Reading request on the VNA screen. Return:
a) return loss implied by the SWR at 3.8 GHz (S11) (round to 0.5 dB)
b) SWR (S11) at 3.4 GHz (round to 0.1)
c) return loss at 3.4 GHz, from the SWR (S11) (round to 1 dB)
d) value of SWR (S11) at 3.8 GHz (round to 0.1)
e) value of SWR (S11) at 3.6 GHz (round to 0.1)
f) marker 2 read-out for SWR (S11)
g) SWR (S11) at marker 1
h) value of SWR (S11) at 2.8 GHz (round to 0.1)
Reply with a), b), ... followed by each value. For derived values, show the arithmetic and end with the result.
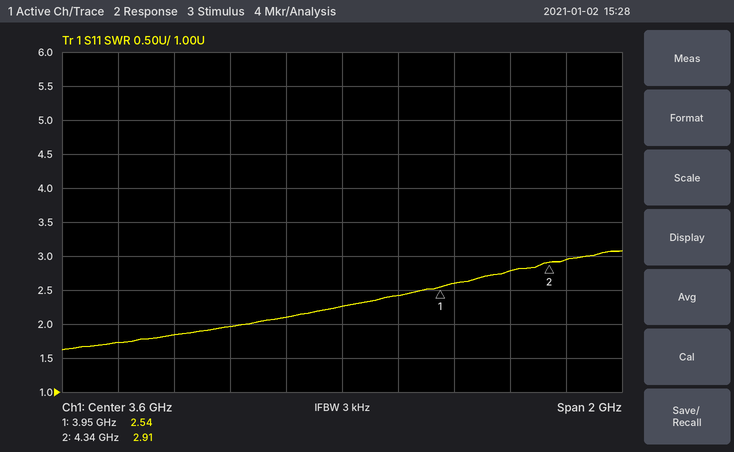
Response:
a) −20 log10((2.4 − 1)/(2.4 + 1)) ≈ 7.71 dB, so 7.5 dB to the nearest 0.5 dB
b) 2.1
c) −20 log10((2.1 − 1)/(2.1 + 1)) ≈ 9 dB
d) 2.4
e) 2.3
f) 2.91
g) 2.54
h) 1.7
